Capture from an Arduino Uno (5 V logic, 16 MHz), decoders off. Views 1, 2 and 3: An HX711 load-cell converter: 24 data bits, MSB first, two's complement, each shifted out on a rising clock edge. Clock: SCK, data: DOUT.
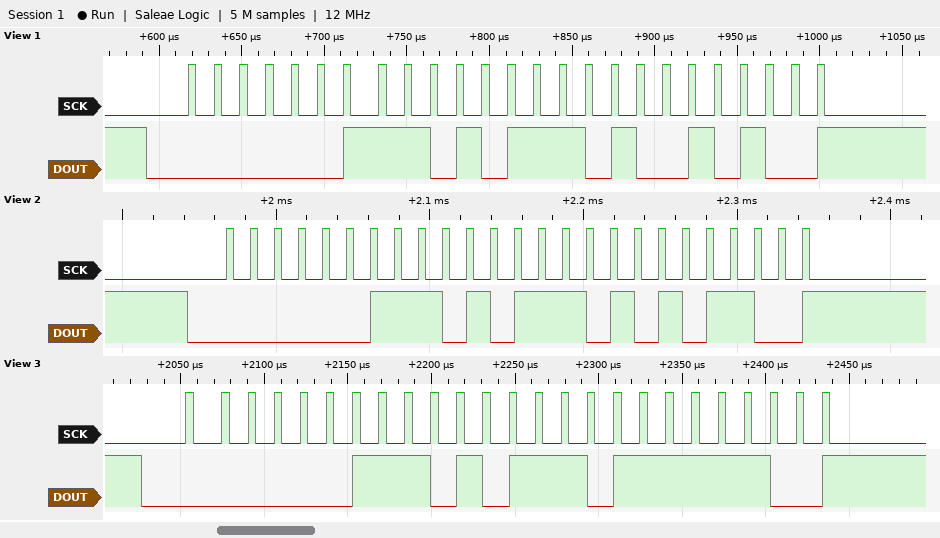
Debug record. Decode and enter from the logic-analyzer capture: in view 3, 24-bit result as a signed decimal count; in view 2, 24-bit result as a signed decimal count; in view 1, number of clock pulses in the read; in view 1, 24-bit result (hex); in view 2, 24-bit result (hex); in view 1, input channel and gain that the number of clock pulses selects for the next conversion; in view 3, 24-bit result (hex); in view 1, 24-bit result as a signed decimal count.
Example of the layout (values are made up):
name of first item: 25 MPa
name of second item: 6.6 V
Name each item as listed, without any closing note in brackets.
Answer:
in view 3, 24-bit result as a signed decimal count: 241404
in view 2, 24-bit result as a signed decimal count: 241324
in view 1, number of clock pulses in the read: 25
in view 1, 24-bit result: 0x03AE94
in view 2, 24-bit result: 0x03AEAC
in view 1, input channel and gain that the number of clock pulses selects for the next conversion: channel A, gain 128
in view 3, 24-bit result: 0x03AEFC
in view 1, 24-bit result as a signed decimal count: 241300
